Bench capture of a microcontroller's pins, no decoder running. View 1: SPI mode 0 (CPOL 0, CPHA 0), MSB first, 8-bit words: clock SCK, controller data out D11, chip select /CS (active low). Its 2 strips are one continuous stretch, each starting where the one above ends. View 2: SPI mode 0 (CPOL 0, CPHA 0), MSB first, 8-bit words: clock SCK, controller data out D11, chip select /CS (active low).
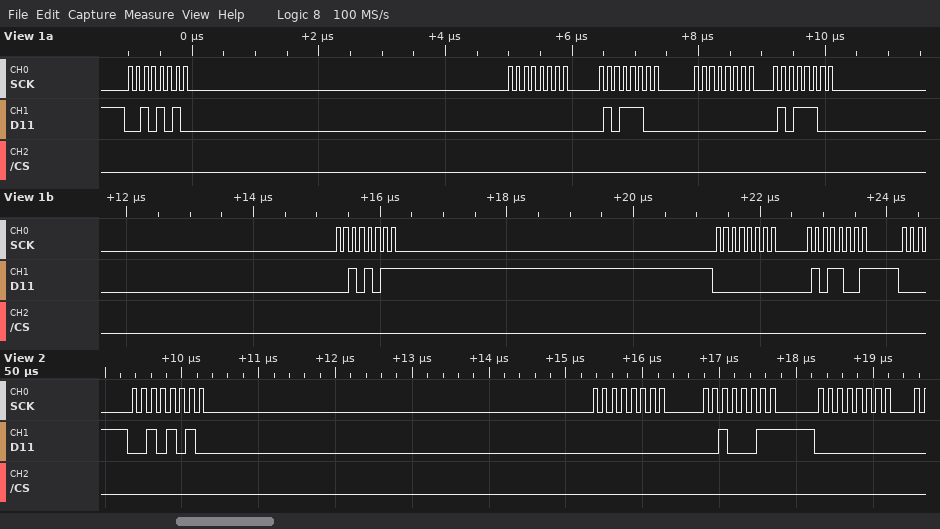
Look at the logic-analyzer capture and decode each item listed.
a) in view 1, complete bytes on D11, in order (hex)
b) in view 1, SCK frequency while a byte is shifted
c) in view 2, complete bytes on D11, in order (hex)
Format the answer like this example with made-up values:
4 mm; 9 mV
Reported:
2A 00 5C 00 5C 2B 00 59; 8 MHz; 2A 00 23 00
